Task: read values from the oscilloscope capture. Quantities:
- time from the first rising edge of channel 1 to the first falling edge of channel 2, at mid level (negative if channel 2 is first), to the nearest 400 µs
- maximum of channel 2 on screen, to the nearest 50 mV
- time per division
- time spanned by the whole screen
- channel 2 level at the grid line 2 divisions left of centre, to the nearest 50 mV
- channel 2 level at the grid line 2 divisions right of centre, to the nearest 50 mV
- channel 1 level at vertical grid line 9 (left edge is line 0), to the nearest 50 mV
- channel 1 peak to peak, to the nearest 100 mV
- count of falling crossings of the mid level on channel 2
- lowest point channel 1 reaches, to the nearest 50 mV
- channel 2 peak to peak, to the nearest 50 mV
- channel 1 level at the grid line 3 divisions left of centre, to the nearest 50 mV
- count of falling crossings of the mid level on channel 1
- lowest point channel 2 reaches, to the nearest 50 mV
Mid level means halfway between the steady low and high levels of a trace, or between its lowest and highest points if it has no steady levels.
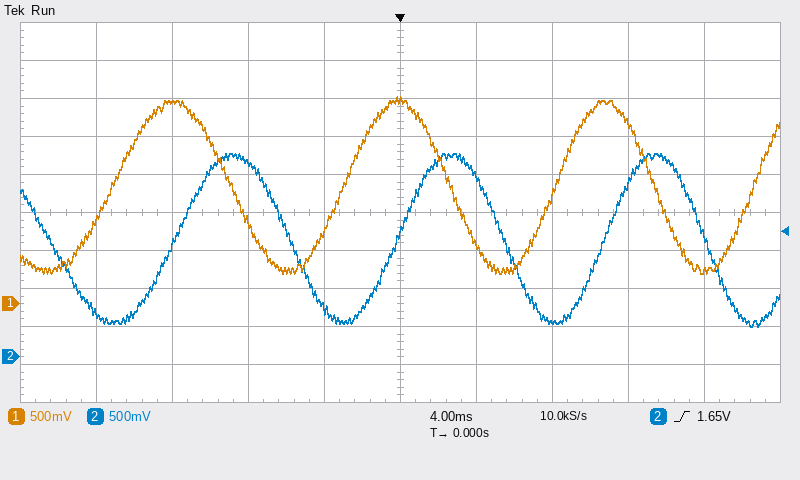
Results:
-3.2 ms
2.70 V
4 ms
40 ms
2.55 V
450 mV
450 mV
2.30 V
4
400 mV
2.30 V
2.65 V
3
400 mV
